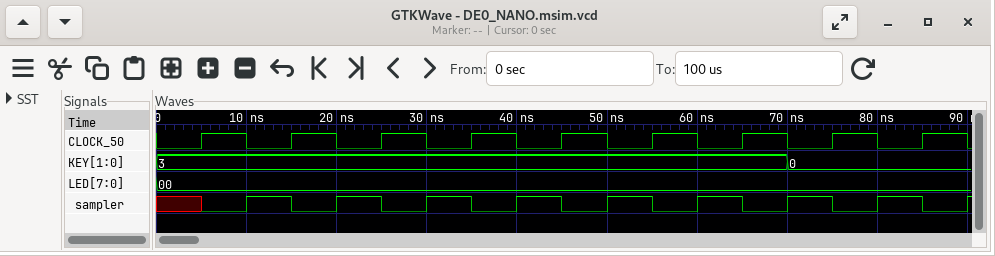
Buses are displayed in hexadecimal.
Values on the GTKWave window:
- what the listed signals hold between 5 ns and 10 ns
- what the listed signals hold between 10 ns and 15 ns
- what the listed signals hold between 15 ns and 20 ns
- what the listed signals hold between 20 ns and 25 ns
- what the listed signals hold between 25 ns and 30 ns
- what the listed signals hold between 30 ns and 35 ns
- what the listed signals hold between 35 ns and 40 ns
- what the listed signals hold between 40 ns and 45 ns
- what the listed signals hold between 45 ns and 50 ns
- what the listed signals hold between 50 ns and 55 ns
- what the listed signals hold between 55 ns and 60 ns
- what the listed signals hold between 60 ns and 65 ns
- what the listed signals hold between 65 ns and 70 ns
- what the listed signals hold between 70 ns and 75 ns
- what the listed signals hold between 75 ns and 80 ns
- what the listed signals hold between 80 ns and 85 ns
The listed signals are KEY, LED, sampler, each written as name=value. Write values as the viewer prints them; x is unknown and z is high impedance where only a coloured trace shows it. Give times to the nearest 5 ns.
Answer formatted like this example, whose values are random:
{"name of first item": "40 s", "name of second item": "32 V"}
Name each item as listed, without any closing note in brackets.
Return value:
{"what the listed signals hold between 5 ns and 10 ns": "KEY=3, LED=00, sampler=0", "what the listed signals hold between 10 ns and 15 ns": "KEY=3, LED=00, sampler=1", "what the listed signals hold between 15 ns and 20 ns": "KEY=3, LED=00, sampler=0", "what the listed signals hold between 20 ns and 25 ns": "KEY=3, LED=00, sampler=1", "what the listed signals hold between 25 ns and 30 ns": "KEY=3, LED=00, sampler=0", "what the listed signals hold between 30 ns and 35 ns": "KEY=3, LED=00, sampler=1", "what the listed signals hold between 35 ns and 40 ns": "KEY=3, LED=00, sampler=0", "what the listed signals hold between 40 ns and 45 ns": "KEY=3, LED=00, sampler=1", "what the listed signals hold between 45 ns and 50 ns": "KEY=3, LED=00, sampler=0", "what the listed signals hold between 50 ns and 55 ns": "KEY=3, LED=00, sampler=1", "what the listed signals hold between 55 ns and 60 ns": "KEY=3, LED=00, sampler=0", "what the listed signals hold between 60 ns and 65 ns": "KEY=3, LED=00, sampler=1", "what the listed signals hold between 65 ns and 70 ns": "KEY=3, LED=00, sampler=0", "what the listed signals hold between 70 ns and 75 ns": "KEY=0, LED=00, sampler=1", "what the listed signals hold between 75 ns and 80 ns": "KEY=0, LED=00, sampler=0", "what the listed signals hold between 80 ns and 85 ns": "KEY=0, LED=00, sampler=1"}
